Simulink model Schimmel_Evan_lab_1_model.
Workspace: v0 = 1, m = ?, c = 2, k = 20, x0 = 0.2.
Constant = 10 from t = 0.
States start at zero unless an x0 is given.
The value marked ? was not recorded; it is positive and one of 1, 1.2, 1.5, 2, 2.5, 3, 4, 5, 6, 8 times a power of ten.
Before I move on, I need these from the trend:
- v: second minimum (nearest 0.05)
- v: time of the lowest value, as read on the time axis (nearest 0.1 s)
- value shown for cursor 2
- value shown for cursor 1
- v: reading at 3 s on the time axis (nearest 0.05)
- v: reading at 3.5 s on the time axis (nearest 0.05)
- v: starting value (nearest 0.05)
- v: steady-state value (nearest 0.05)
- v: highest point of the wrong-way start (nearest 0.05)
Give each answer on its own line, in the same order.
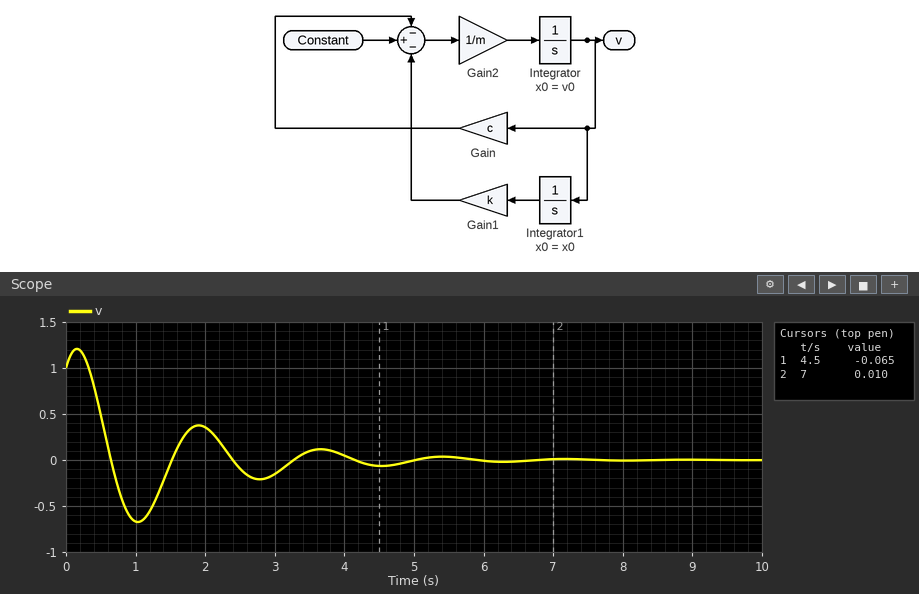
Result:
-0.20
1.0 s
0.010
-0.065
-0.15
0.10
1.00
0.00
1.20
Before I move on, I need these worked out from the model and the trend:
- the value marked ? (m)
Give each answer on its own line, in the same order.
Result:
1.5
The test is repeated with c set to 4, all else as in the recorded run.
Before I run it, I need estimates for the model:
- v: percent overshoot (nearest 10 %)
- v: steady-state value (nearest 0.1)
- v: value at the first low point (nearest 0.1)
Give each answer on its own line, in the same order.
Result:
30 %
0.0
-0.3
